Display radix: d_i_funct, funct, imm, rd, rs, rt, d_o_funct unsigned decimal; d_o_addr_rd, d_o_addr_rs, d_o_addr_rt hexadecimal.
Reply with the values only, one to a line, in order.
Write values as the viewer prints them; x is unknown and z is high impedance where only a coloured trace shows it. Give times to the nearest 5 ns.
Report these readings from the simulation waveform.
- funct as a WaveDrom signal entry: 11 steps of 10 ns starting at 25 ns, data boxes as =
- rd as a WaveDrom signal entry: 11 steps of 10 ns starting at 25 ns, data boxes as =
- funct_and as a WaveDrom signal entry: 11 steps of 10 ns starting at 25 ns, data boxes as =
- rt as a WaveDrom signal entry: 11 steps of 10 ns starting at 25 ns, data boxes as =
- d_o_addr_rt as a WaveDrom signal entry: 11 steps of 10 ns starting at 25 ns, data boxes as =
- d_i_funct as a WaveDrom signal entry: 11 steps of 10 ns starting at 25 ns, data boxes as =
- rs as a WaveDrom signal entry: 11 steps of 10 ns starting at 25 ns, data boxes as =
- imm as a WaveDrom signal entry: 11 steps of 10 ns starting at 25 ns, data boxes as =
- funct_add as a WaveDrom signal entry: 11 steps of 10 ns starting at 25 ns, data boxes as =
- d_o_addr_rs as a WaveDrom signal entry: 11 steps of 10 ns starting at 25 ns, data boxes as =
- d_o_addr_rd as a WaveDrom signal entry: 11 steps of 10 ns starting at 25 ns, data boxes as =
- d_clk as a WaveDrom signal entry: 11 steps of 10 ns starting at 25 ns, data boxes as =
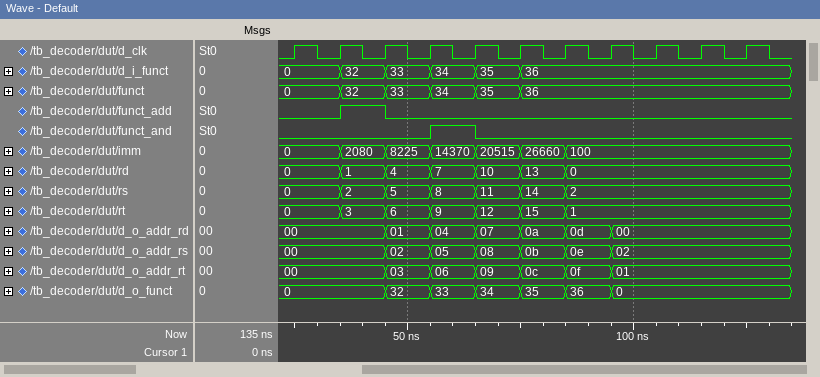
{name: 'funct', wave: '======.....', data: '0 32 33 34 35 36'}
{name: 'rd', wave: '=======....', data: '0 1 4 7 10 13 0'}
{name: 'funct_and', wave: '0..10......'}
{name: 'rt', wave: '=======....', data: '0 3 6 9 12 15 1'}
{name: 'd_o_addr_rt', wave: '=.======...', data: '00 03 06 09 0c 0f 01'}
{name: 'd_i_funct', wave: '======.....', data: '0 32 33 34 35 36'}
{name: 'rs', wave: '=======....', data: '0 2 5 8 11 14 2'}
{name: 'imm', wave: '=======....', data: '0 2080 8225 14370 20515 26660 100'}
{name: 'funct_add', wave: '010........'}
{name: 'd_o_addr_rs', wave: '=.======...', data: '00 02 05 08 0b 0e 02'}
{name: 'd_o_addr_rd', wave: '=.======...', data: '00 01 04 07 0a 0d 00'}
{name: 'd_clk', wave: 'p..........'}
